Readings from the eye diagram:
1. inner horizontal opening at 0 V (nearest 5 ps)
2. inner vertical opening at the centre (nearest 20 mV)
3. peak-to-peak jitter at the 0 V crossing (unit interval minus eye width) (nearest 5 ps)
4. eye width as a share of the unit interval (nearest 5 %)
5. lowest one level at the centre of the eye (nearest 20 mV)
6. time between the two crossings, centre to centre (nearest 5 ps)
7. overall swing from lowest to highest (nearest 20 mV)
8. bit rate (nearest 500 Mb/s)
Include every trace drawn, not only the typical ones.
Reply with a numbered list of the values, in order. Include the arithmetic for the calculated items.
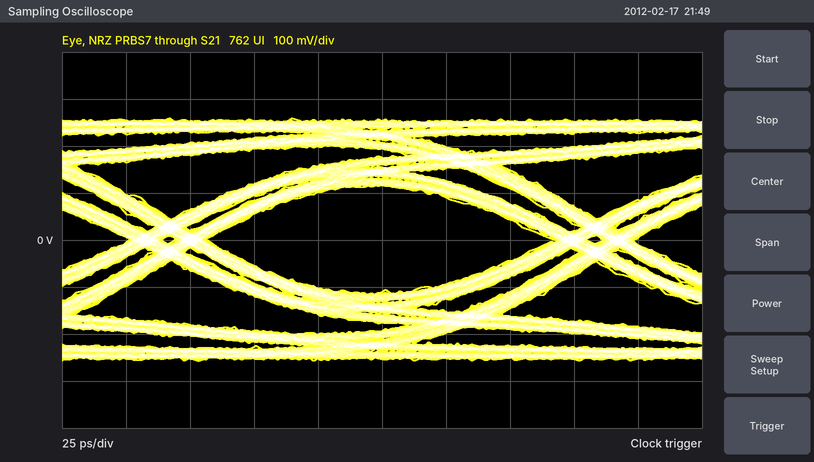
1. 135 ps
2. 220 mV
3. 30 ps
4. 135 ps / 165 ps ≈ 81.8 %, so 80 % to the nearest 5 %
5. 120 mV
6. 165 ps
7. 520 mV
8. 6.0 Gb/s
